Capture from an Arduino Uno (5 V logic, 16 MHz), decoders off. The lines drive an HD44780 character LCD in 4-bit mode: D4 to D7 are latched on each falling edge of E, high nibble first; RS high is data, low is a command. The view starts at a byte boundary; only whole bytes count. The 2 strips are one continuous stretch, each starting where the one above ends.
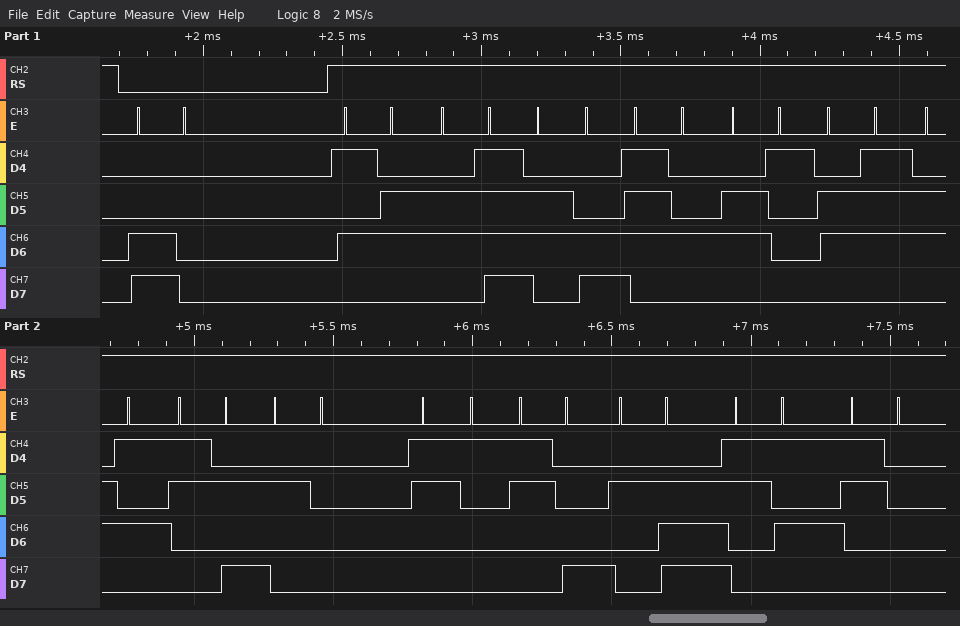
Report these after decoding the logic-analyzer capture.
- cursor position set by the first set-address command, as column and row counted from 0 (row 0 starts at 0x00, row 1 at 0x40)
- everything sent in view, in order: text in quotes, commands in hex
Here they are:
column 0, row 1
0xC0 "Voltage: 18.50"
